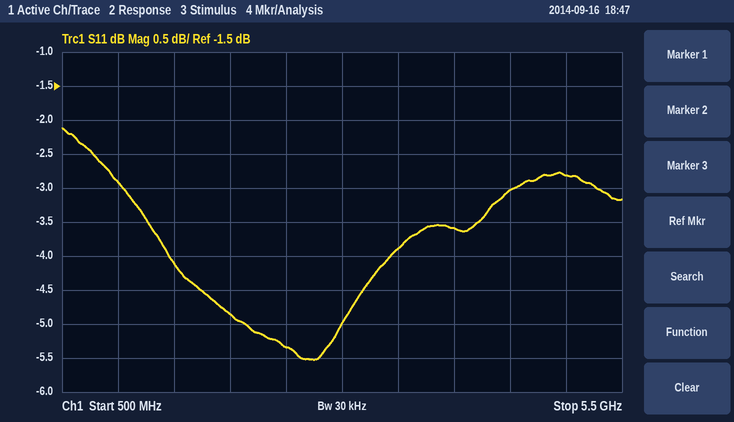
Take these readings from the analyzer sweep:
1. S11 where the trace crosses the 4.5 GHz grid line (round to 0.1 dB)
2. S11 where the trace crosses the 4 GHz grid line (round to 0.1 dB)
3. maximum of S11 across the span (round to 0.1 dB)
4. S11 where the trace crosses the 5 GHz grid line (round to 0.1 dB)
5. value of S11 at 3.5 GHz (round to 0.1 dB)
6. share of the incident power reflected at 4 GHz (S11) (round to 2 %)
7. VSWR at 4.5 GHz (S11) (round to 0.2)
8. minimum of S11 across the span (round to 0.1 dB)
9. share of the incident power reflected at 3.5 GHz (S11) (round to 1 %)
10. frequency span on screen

-3.0 dB
-3.6 dB
-2.1 dB
-2.8 dB
-3.9 dB
44 %
5.8
-5.5 dB
41 %
5 GHz
